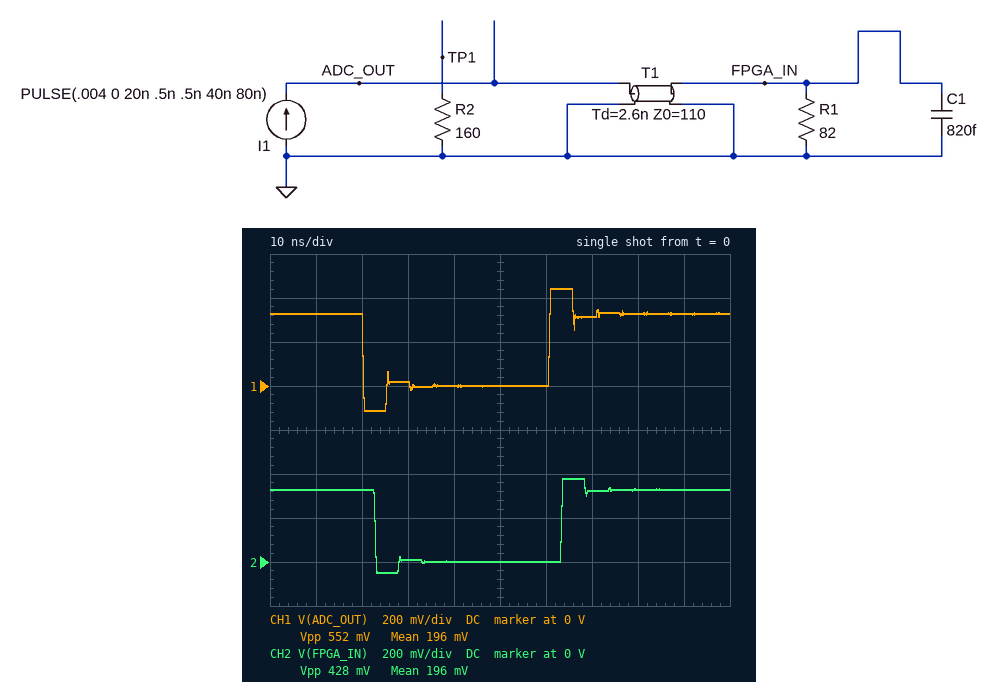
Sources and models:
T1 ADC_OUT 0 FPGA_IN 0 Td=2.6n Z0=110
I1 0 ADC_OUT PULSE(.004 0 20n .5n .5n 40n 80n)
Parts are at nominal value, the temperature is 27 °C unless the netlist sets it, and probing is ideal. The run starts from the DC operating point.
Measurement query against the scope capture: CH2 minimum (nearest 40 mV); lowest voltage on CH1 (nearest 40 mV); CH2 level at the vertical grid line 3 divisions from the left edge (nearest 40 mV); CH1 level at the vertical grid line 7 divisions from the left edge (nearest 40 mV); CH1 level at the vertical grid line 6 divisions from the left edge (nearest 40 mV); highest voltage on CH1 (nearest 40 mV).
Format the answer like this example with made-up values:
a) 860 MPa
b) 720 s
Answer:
a) -40 mV
b) -120 mV
c) 0 V
d) 320 mV
e) 0 V
f) 440 mV
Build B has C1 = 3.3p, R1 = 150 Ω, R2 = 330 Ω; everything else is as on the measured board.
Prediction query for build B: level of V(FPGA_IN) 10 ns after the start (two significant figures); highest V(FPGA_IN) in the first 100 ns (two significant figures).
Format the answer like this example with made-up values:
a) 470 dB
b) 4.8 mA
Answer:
a) 600 mV
b) 640 mV
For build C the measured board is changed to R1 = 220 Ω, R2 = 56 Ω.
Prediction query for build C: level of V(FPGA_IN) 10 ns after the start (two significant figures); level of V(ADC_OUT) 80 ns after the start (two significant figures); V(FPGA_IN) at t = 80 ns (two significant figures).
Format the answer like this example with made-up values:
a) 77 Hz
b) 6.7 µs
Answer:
a) 880 mV
b) 860 mV
c) 870 mV
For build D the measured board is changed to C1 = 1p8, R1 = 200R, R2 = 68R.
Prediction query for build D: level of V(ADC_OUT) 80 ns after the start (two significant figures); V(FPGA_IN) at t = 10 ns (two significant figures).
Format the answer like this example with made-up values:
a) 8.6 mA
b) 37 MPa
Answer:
a) 790 mV
b) 800 mV
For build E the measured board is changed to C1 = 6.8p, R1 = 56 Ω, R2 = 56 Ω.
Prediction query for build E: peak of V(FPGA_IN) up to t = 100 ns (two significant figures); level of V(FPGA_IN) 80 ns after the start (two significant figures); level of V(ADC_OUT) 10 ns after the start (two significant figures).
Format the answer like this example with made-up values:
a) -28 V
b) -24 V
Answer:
a) 310 mV
b) 230 mV
c) 220 mV
